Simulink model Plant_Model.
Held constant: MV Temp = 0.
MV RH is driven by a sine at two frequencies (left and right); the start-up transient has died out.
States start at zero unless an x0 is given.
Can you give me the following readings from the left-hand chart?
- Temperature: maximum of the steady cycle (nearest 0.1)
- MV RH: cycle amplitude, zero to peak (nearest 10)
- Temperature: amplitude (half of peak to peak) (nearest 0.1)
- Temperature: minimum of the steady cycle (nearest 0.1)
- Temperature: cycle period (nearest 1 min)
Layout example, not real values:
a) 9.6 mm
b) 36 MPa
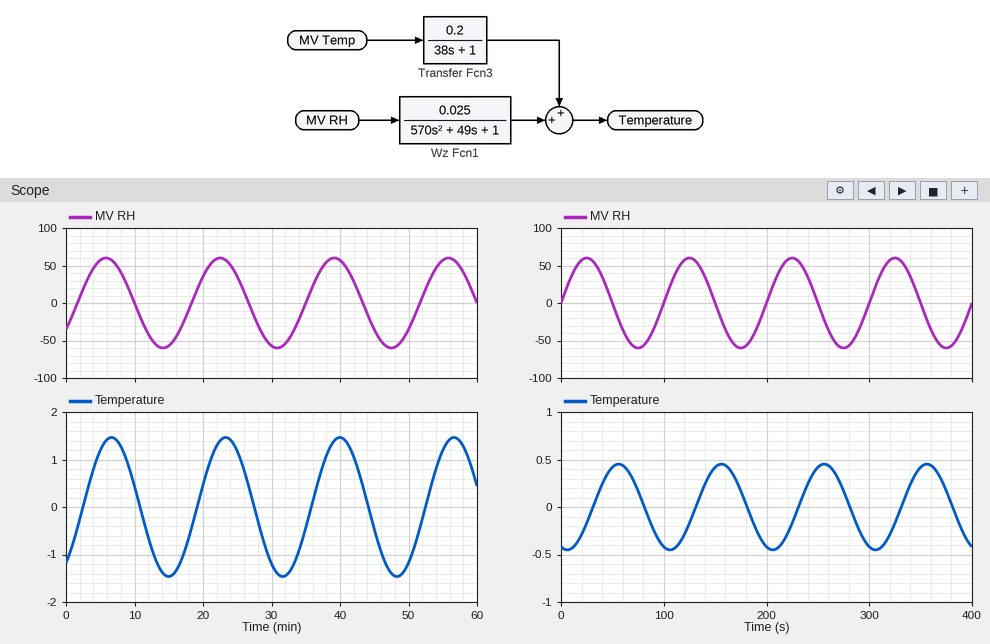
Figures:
a) 1.5
b) 60
c) 1.5
d) -1.5
e) 17 min
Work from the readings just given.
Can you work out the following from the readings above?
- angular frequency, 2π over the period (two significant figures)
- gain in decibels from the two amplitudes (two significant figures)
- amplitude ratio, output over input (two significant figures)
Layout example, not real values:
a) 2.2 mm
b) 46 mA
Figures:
a) 0.37 rad/min
b) -32 dB
c) 0.025
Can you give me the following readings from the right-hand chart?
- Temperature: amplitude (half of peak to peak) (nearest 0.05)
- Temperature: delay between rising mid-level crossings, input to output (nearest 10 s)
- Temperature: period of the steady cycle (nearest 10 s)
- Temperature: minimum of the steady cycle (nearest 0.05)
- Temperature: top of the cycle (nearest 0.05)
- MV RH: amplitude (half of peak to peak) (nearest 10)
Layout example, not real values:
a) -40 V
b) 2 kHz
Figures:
a) 0.45
b) 30 s
c) 100 s
d) -0.45
e) 0.45
f) 60
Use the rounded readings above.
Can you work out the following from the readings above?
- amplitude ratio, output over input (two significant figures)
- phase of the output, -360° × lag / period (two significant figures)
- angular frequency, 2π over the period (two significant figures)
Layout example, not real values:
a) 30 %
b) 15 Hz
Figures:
a) 0.0075
b) -110°
c) 0.063 rad/s
